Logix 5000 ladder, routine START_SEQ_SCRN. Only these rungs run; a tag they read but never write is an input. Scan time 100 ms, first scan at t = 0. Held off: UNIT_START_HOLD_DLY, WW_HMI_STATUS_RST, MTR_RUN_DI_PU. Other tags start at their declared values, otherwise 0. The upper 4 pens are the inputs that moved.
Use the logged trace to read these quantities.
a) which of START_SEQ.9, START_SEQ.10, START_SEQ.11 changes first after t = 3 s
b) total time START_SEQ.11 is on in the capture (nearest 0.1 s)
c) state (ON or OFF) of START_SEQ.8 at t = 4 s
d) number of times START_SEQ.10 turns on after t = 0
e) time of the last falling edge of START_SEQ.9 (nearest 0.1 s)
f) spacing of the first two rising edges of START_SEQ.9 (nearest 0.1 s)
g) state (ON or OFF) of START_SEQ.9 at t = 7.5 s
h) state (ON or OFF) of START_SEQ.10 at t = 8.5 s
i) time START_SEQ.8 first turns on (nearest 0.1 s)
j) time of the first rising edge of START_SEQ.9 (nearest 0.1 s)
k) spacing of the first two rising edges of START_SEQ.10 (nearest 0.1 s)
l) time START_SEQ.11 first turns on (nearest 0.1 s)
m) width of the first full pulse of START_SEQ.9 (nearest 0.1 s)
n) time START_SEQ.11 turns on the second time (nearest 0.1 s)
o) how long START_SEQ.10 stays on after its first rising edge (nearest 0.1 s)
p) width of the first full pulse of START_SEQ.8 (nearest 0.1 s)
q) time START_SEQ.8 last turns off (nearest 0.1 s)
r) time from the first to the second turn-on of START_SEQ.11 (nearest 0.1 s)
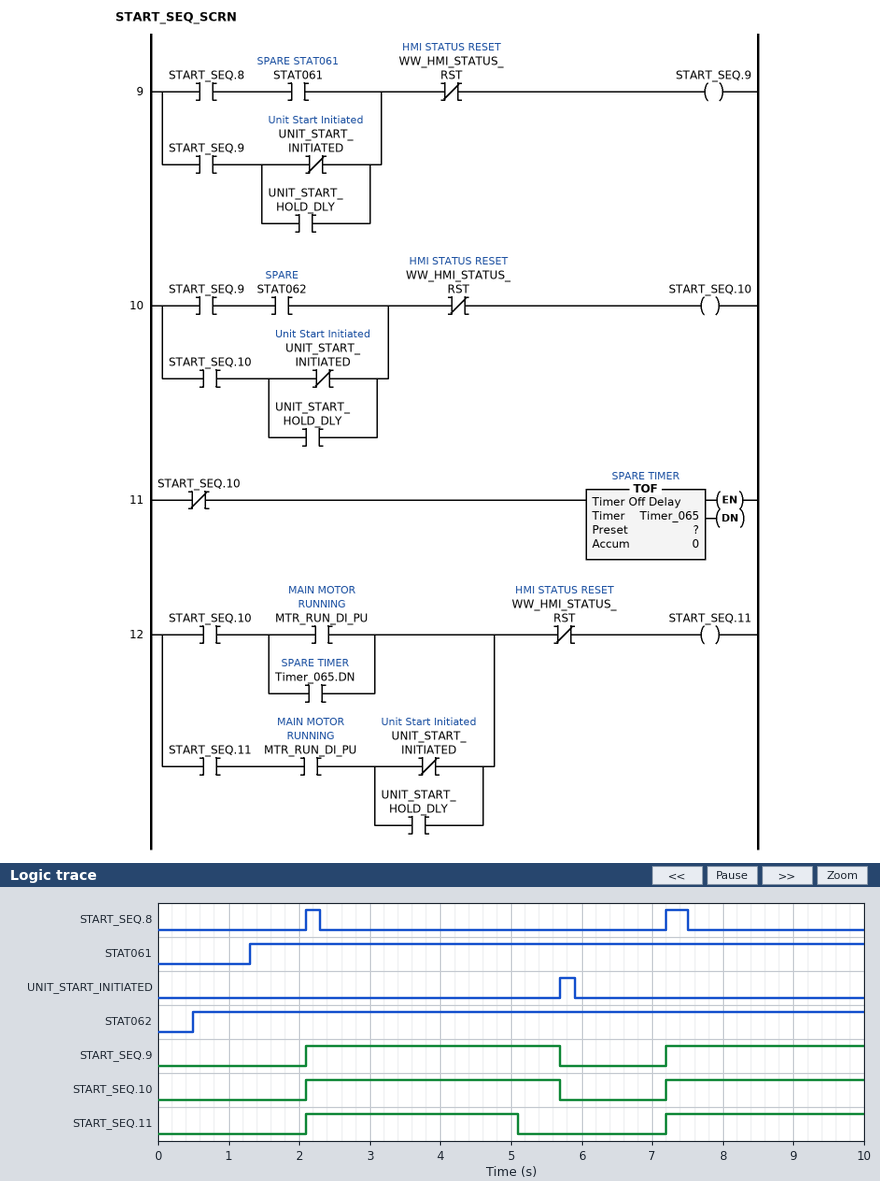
START_SEQ.11
5.8 s
OFF
2
5.7 s
5.1 s
ON
ON
2.1 s
2.1 s
5.1 s
2.1 s
3.6 s
7.2 s
3.6 s
0.2 s
7.5 s
5.1 s
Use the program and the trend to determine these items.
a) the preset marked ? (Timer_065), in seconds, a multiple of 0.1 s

3.0 s
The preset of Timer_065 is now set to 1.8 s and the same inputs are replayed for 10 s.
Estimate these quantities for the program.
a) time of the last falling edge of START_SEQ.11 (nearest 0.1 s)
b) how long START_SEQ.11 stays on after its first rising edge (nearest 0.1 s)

9.0 s
1.8 s
